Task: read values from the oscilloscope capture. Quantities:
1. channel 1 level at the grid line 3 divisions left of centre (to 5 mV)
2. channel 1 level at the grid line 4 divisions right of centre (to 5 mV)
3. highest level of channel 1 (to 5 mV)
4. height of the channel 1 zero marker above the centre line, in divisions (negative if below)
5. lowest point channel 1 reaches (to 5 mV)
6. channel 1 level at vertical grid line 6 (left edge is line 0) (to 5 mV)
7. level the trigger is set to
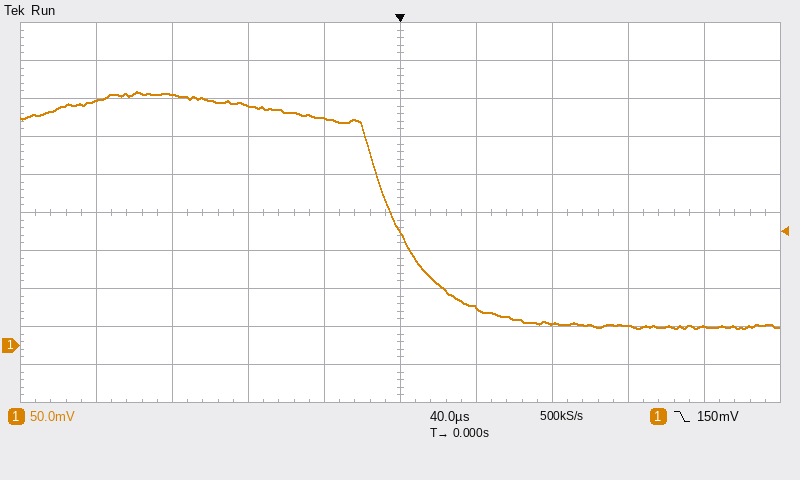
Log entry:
330 mV
25 mV
335 mV
-3.5 div
20 mV
50 mV
150 mV
